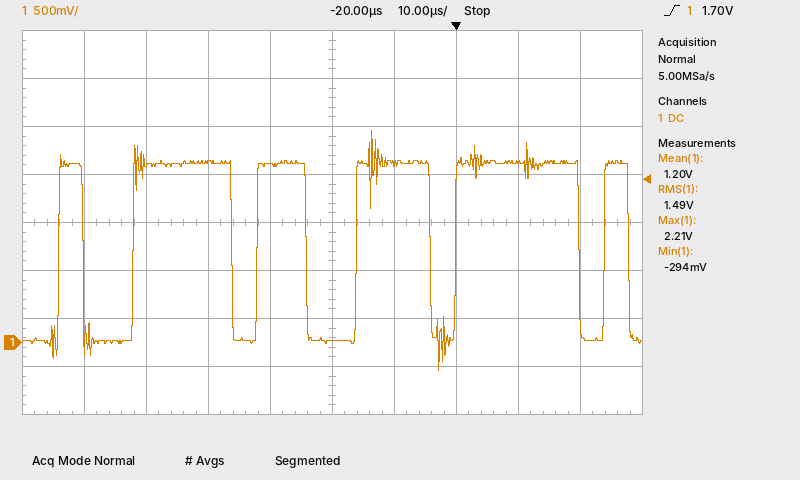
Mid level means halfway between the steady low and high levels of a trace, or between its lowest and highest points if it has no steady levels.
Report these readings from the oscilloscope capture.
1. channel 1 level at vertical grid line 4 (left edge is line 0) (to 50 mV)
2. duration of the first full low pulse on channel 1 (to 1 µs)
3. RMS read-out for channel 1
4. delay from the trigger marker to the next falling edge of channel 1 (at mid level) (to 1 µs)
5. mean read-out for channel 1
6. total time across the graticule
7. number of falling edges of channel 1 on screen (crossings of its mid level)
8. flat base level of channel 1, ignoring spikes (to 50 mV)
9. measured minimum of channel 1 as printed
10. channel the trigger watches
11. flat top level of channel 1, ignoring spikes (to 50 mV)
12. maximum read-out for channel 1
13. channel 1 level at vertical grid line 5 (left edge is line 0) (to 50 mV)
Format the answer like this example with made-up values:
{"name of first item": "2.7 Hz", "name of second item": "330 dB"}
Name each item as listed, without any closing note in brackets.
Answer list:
{"channel 1 level at vertical grid line 4 (left edge is line 0)": "1.85 V", "duration of the first full low pulse on channel 1": "8 µs", "RMS read-out for channel 1": "1.49 V", "delay from the trigger marker to the next falling edge of channel 1 (at mid level)": "20 µs", "mean read-out for channel 1": "1.20 V", "total time across the graticule": "100 µs", "number of falling edges of channel 1 on screen": "6", "flat base level of channel 1, ignoring spikes": "0 mV", "measured minimum of channel 1 as printed": "-294 mV", "channel the trigger watches": "channel 1", "flat top level of channel 1, ignoring spikes": "1.85 V", "maximum read-out for channel 1": "2.21 V", "channel 1 level at vertical grid line 5 (left edge is line 0)": "0 mV"}
